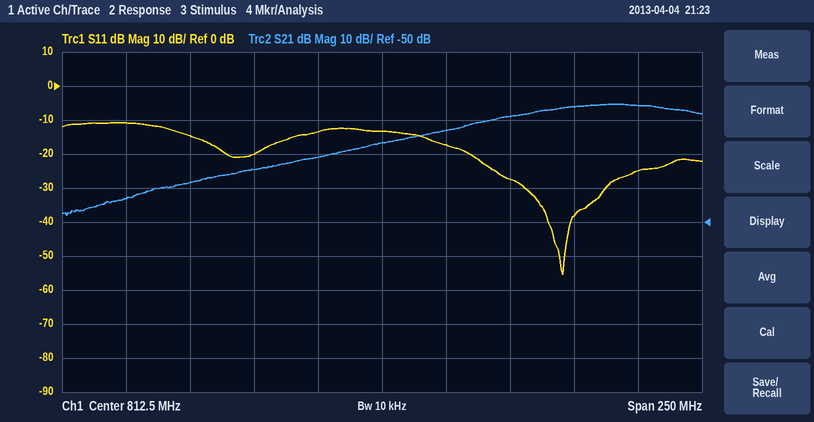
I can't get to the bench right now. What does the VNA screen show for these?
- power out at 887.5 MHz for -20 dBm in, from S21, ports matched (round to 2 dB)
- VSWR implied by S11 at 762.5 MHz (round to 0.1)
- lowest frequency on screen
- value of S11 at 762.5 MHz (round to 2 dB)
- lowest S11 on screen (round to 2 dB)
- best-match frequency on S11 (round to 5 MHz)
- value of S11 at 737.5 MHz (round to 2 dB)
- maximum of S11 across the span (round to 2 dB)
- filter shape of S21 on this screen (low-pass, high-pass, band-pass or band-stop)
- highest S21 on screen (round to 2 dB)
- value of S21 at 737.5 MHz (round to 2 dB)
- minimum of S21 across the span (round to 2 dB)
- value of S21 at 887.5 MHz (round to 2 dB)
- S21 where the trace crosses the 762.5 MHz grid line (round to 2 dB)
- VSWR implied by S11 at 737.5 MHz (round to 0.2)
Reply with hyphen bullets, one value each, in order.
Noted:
- -36 dBm
- 1.2
- 687.5 MHz
- -20 dB
- -56 dB
- 885 MHz
- -14 dB
- -10 dB
- high-pass
- -16 dB
- -38 dB
- -48 dB
- -16 dB
- -34 dB
- 1.4
